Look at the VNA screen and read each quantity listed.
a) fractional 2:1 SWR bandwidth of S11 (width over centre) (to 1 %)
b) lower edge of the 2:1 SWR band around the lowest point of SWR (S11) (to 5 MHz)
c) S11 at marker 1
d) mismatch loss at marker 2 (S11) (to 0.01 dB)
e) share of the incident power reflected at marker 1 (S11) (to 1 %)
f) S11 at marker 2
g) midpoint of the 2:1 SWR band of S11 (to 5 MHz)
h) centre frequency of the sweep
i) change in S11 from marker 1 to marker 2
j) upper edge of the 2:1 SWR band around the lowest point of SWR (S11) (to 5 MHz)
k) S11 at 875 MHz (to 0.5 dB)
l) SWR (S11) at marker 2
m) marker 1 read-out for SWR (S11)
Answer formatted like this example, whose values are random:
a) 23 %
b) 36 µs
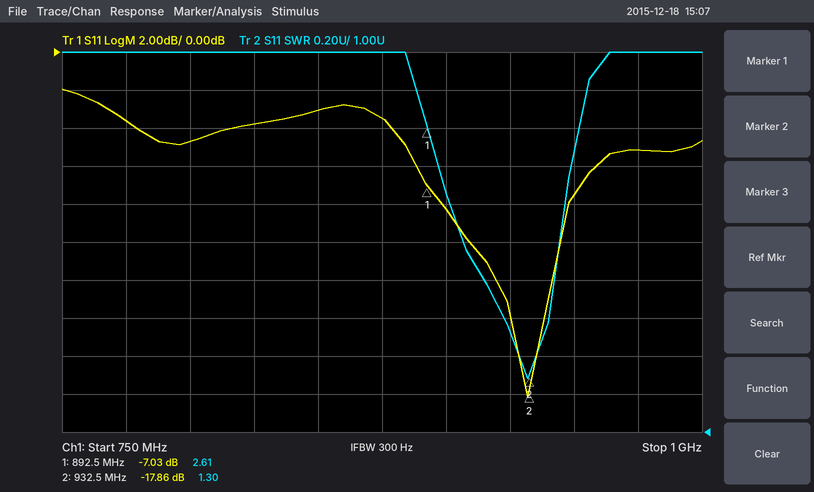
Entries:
a) 4 %
b) 905 MHz
c) -7.03 dB
d) 0.07 dB
e) 20 %
f) -17.86 dB
g) 925 MHz
h) 875 MHz
i) -10.83 dB
j) 945 MHz
k) -3.5 dB
l) 1.30
m) 2.61
